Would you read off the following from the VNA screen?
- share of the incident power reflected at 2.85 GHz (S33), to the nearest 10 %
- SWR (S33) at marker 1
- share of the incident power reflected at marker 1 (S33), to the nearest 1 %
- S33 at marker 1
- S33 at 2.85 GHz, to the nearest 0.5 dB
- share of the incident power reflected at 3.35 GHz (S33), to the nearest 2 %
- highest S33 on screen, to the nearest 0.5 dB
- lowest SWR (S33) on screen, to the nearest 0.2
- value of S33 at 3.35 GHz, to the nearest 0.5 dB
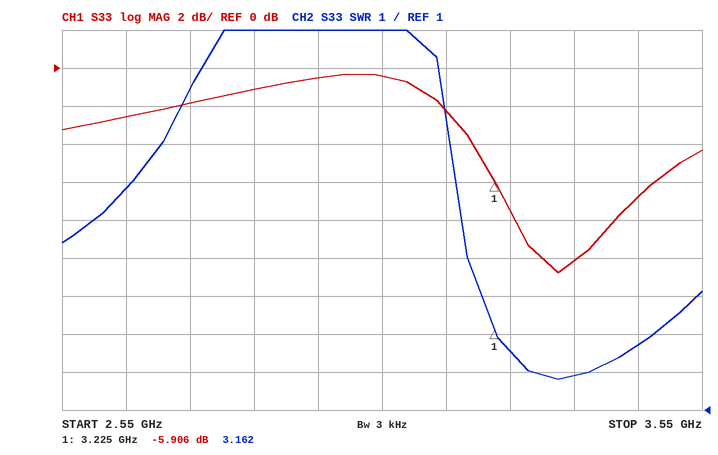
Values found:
80 %
3.162
26 %
-5.906 dB
-1.0 dB
10 %
-0.5 dB
1.8
-10.0 dB
